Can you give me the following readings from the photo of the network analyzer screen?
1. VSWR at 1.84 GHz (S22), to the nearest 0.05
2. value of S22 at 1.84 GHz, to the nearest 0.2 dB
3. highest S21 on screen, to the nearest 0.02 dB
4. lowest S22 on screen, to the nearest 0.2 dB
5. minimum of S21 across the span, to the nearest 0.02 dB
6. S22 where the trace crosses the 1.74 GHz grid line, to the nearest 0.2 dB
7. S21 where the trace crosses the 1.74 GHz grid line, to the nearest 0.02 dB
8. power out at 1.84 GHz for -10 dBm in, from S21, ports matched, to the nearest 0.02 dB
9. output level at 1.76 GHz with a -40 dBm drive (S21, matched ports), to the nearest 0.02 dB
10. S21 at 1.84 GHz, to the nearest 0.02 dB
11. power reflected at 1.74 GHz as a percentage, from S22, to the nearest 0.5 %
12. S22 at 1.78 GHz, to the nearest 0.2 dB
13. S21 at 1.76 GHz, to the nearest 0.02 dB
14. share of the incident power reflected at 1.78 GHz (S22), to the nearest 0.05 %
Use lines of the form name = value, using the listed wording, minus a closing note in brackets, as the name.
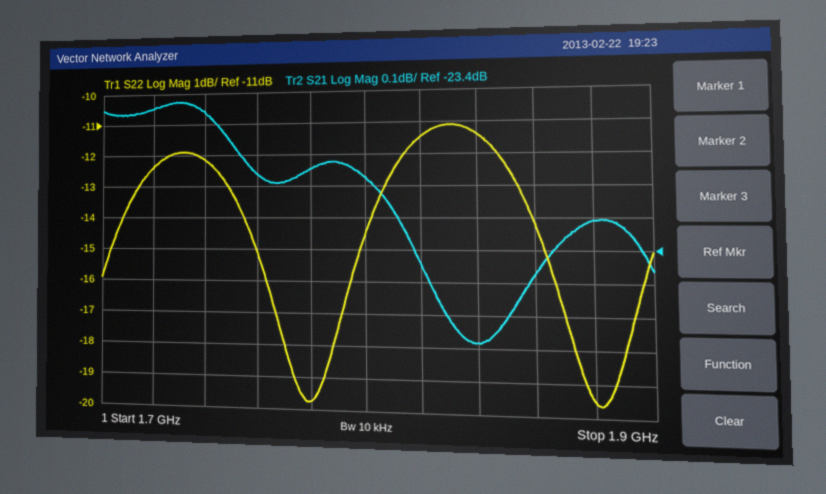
VSWR at 1.84 GHz (S22), to the nearest 0.05 = 1.75
value of S22 at 1.84 GHz, to the nearest 0.2 dB = -11.4 dB
highest S21 on screen, to the nearest 0.02 dB = -22.92 dB
lowest S22 on screen, to the nearest 0.2 dB = -19.8 dB
minimum of S21 across the span, to the nearest 0.02 dB = -23.68 dB
S22 where the trace crosses the 1.74 GHz grid line, to the nearest 0.2 dB = -12.2 dB
S21 where the trace crosses the 1.74 GHz grid line, to the nearest 0.02 dB = -22.96 dB
power out at 1.84 GHz for -10 dBm in, from S21, ports matched, to the nearest 0.02 dB = -33.68 dBm
output level at 1.76 GHz with a -40 dBm drive (S21, matched ports), to the nearest 0.02 dB = -63.16 dBm
S21 at 1.84 GHz, to the nearest 0.02 dB = -23.68 dB
power reflected at 1.74 GHz as a percentage, from S22, to the nearest 0.5 % = 6.0 %
S22 at 1.78 GHz, to the nearest 0.2 dB = -19.8 dB
S21 at 1.76 GHz, to the nearest 0.02 dB = -23.16 dB
share of the incident power reflected at 1.78 GHz (S22), to the nearest 0.05 % = 1.05 %
